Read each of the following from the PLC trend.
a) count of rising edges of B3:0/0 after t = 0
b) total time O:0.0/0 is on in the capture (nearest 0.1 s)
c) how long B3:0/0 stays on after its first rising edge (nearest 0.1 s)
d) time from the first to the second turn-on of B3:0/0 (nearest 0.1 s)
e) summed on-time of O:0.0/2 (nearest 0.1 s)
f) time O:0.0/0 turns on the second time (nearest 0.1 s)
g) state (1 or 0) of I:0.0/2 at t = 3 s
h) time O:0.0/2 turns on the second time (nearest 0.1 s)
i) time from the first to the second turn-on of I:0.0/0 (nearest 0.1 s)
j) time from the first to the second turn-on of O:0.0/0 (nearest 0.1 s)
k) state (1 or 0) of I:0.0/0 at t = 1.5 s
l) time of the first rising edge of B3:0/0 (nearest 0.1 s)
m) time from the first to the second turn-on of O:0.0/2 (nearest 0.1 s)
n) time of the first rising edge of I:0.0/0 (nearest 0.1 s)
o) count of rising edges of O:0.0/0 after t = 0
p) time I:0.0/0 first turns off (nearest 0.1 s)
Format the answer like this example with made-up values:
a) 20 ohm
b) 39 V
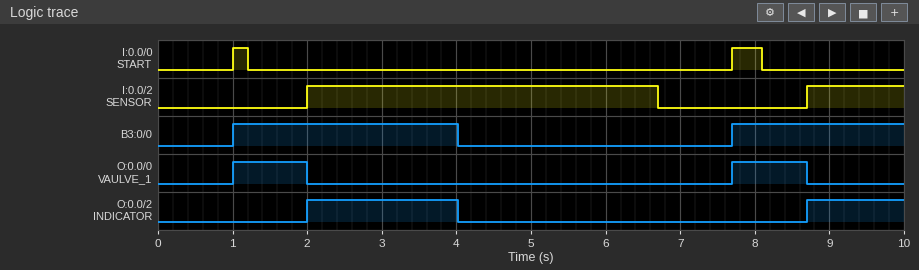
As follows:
a) 2
b) 2.0 s
c) 3.0 s
d) 6.7 s
e) 3.3 s
f) 7.7 s
g) 1
h) 8.7 s
i) 6.7 s
j) 6.7 s
k) 0
l) 1.0 s
m) 6.7 s
n) 1.0 s
o) 2
p) 1.2 s
